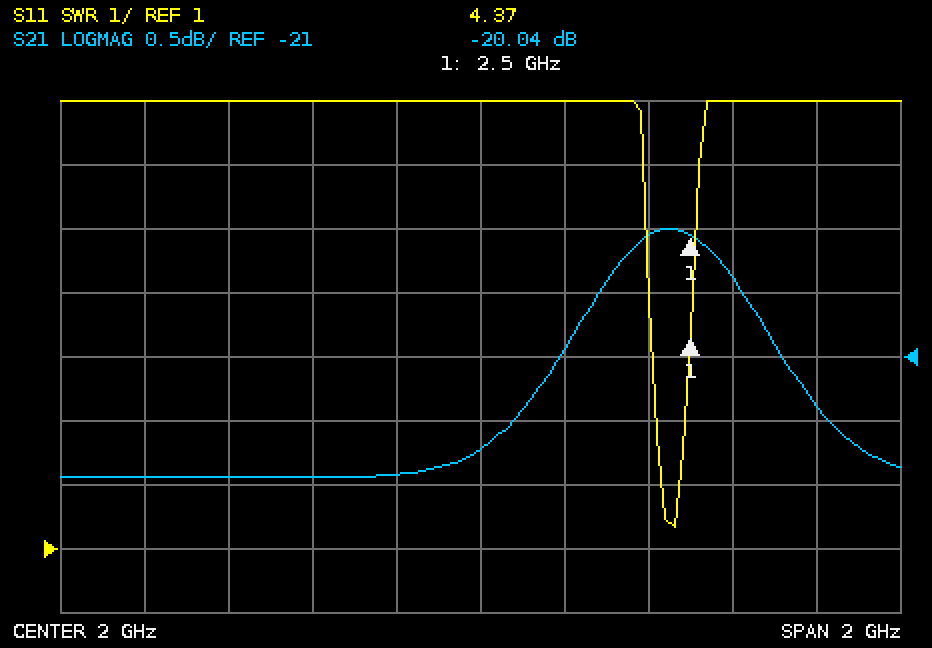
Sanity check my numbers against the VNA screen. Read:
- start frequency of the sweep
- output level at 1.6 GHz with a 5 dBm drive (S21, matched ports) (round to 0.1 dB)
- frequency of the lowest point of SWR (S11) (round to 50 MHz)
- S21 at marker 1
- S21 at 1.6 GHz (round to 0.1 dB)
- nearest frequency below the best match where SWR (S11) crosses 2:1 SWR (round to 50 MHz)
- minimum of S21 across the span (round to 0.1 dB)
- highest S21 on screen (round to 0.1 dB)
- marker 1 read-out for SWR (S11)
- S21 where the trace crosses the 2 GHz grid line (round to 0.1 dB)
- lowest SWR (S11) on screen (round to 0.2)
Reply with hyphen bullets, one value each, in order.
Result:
- 1 GHz
- -16.9 dBm
- 2.45 GHz
- -20.04 dB
- -21.9 dB
- 2.45 GHz
- -21.9 dB
- -20.0 dB
- 4.37
- -21.7 dB
- 1.4
